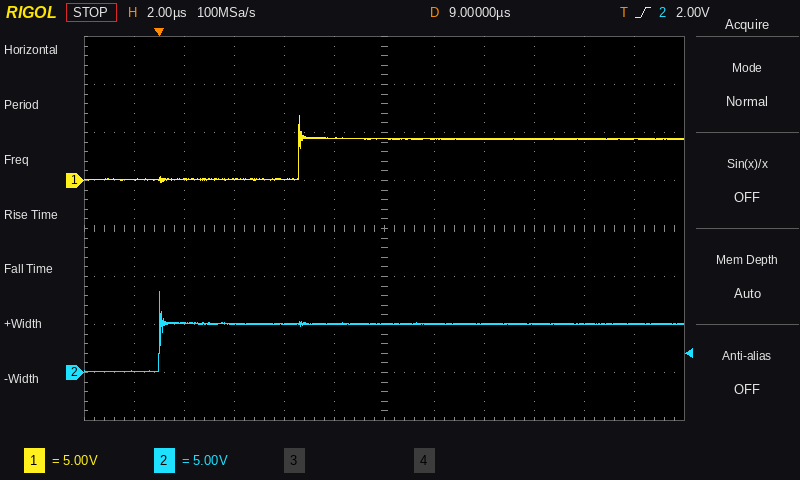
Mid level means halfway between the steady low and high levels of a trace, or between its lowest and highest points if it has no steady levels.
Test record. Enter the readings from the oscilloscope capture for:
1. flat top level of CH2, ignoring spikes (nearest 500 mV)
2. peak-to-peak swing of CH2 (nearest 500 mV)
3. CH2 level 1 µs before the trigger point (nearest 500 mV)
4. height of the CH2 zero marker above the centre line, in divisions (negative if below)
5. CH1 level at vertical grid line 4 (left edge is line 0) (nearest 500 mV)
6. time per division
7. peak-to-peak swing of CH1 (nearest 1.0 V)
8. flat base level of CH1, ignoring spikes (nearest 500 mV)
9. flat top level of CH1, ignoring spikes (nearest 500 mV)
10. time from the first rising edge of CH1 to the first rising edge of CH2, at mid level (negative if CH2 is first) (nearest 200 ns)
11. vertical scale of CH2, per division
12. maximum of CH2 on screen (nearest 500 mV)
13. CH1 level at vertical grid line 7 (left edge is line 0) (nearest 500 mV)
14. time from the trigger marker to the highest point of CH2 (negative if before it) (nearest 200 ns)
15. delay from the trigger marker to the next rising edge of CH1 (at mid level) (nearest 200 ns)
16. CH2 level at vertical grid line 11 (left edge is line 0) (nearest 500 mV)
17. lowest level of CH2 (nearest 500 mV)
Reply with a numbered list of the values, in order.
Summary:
1. 5.0 V
2. 8.5 V
3. 0.0 V
4. -3.0 div
5. 0.0 V
6. 2 µs
7. 7.0 V
8. 0.0 V
9. 4.5 V
10. -5.6 µs
11. 5 V
12. 8.5 V
13. 4.5 V
14. 0.0 µs
15. 5.6 µs
16. 5.0 V
17. 0.0 V
